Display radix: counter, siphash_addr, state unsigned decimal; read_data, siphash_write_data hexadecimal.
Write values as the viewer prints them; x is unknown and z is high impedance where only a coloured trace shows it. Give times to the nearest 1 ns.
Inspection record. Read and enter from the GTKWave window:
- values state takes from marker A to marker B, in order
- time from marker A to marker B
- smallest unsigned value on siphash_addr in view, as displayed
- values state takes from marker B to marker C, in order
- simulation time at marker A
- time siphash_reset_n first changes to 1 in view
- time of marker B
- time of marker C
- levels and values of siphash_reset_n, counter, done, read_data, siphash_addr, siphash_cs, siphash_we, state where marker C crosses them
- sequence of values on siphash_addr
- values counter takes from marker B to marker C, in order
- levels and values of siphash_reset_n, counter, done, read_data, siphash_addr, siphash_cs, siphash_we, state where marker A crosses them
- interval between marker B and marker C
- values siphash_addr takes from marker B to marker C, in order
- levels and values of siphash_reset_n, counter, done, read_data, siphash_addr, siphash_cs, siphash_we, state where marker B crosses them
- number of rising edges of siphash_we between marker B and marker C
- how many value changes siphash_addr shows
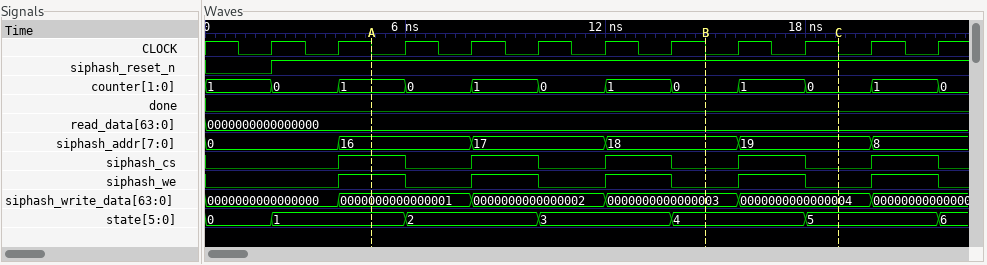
1, 2, 3, 4
10 ns
0
4, 5
5 ns
2 ns
15 ns
19 ns
siphash_reset_n=1, counter=0, done=0, read_data=0000000000000000, siphash_addr=19, siphash_cs=0, siphash_we=0, state=5
0, 16, 17, 18, 19, 8
0, 1, 0
siphash_reset_n=1, counter=1, done=0, read_data=0000000000000000, siphash_addr=16, siphash_cs=1, siphash_we=1, state=1
4 ns
18, 19
siphash_reset_n=1, counter=0, done=0, read_data=0000000000000000, siphash_addr=18, siphash_cs=0, siphash_we=0, state=4
1
5
